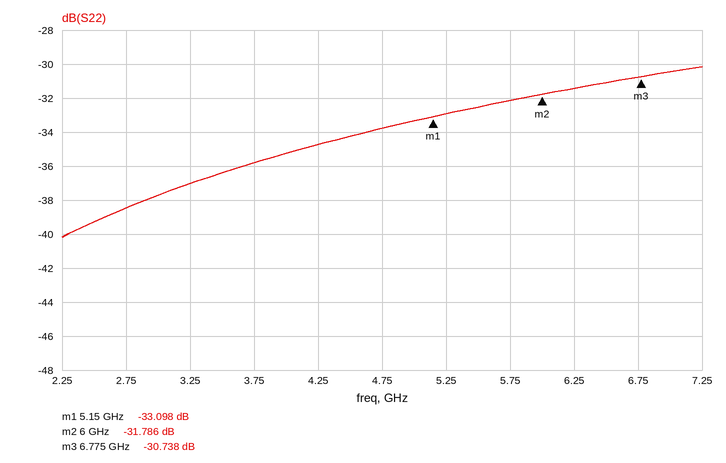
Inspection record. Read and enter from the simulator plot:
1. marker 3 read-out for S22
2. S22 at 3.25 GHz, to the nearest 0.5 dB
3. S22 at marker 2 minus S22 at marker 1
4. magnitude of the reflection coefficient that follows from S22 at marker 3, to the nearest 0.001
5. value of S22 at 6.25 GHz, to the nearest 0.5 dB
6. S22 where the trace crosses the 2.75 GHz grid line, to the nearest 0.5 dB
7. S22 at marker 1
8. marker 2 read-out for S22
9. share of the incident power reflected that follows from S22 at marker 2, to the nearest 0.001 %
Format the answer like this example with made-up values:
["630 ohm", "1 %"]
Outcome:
["-30.738 dB", "-37.0 dB", "1.312 dB", "0.029", "-31.5 dB", "-38.5 dB", "-33.098 dB", "-31.786 dB", "0.066 %"]
